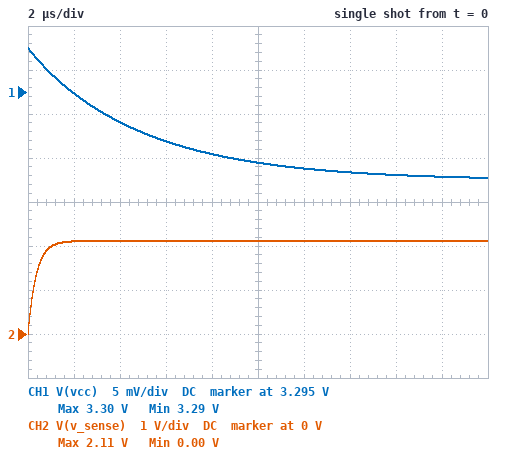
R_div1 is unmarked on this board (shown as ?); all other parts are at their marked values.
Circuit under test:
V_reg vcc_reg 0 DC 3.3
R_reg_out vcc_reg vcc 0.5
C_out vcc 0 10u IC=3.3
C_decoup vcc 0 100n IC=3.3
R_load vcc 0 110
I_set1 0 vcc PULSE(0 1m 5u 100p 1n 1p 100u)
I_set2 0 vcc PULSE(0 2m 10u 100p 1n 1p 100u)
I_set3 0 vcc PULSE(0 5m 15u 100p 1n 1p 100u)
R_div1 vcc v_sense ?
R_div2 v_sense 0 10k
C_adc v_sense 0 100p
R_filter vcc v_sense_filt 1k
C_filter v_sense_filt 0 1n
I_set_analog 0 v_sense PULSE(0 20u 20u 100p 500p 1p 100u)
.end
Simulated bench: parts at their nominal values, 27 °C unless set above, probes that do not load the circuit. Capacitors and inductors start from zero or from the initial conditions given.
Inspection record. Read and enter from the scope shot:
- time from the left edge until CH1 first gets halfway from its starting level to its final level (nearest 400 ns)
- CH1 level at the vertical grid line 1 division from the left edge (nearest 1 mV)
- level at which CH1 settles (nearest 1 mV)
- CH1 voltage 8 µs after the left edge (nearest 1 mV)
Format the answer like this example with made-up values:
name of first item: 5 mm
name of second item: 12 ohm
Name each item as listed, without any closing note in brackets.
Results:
time from the left edge until CH1 first gets halfway from its starting level to its final level: 3.2 µs
CH1 level at the vertical grid line 1 division from the left edge: 3.295 V
level at which CH1 settles: 3.285 V
CH1 voltage 8 µs after the left edge: 3.288 V
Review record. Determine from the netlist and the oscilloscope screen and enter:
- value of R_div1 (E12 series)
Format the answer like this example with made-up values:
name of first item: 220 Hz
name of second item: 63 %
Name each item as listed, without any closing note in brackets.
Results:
value of R_div1: 5.6 kΩ
